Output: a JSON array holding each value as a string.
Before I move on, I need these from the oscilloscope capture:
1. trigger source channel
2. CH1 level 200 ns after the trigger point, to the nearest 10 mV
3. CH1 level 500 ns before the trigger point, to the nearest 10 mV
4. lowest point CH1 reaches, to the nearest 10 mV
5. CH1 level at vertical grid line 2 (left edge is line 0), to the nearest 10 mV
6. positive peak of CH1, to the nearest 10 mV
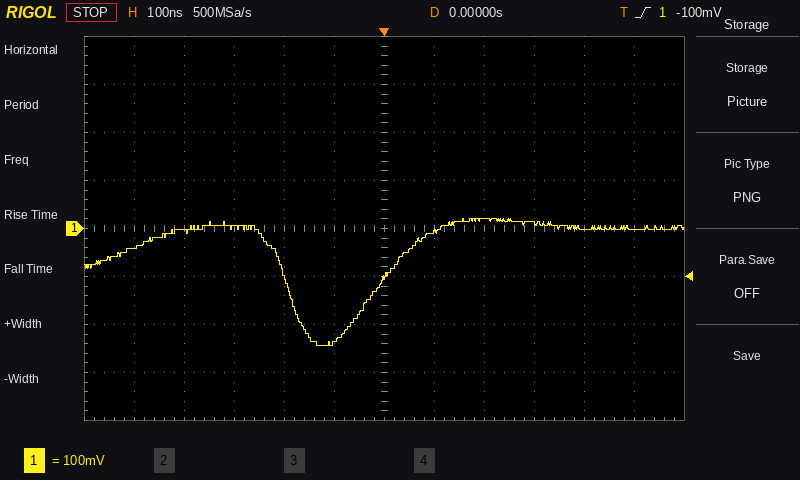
["CH1", "20 mV", "-40 mV", "-240 mV", "-10 mV", "20 mV"]
